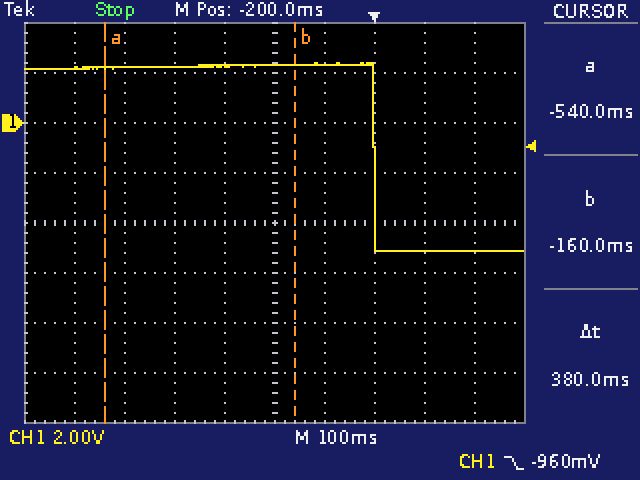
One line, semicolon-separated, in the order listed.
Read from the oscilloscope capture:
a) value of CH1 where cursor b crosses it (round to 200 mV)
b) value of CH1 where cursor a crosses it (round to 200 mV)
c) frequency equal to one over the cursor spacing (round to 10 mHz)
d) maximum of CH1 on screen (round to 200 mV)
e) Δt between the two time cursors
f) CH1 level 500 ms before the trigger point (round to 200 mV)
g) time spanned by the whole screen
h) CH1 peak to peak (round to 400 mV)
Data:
2.4 V; 2.2 V; 2.63 Hz; 2.4 V; 380 ms; 2.2 V; 1 s; 7.6 V
